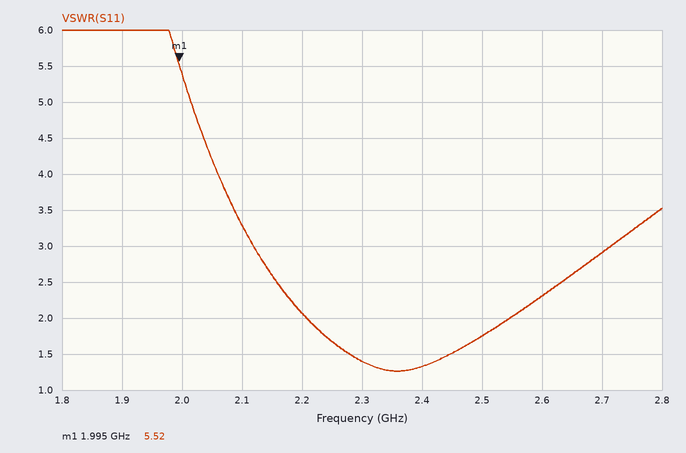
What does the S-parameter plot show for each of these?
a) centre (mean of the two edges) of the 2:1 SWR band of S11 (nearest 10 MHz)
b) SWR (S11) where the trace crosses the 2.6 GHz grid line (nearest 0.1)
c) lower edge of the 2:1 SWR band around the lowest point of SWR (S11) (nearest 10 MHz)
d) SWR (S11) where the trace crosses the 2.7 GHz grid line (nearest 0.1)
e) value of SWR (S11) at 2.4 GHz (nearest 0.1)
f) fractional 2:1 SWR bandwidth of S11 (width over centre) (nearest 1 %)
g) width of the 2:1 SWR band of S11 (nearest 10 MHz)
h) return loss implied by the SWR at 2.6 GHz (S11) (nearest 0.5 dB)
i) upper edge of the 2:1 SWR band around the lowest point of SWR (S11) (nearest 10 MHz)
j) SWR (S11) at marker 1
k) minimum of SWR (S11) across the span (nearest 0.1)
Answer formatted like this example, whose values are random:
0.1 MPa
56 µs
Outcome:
2.38 GHz
2.3
2.21 GHz
2.9
1.3
14 %
340 MHz
8.0 dB
2.55 GHz
5.52
1.3
